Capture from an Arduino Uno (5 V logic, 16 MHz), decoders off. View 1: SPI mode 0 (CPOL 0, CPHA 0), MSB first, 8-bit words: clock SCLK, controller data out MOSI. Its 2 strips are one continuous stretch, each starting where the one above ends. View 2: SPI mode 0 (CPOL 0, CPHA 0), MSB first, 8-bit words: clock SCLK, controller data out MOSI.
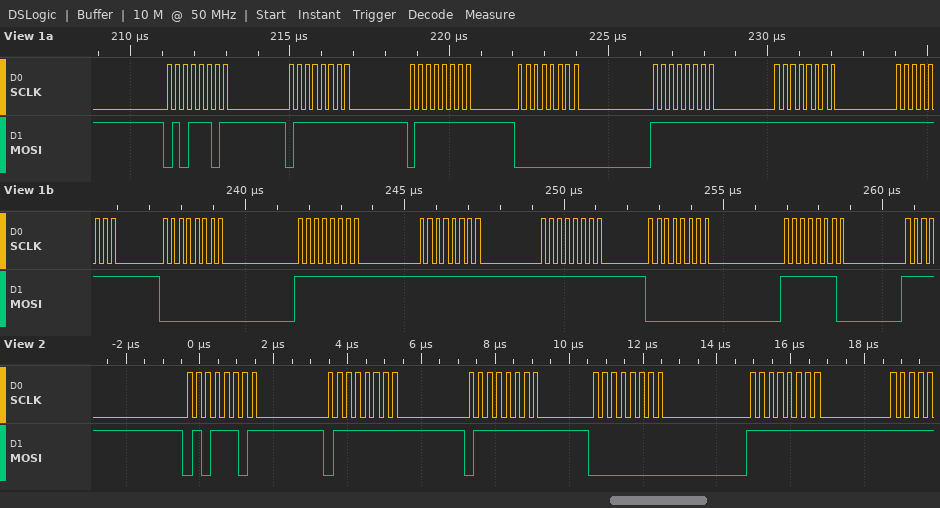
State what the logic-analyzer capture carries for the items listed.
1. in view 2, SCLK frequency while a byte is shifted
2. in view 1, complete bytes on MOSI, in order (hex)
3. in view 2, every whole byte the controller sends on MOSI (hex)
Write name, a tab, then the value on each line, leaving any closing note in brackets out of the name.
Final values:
in view 2, SCLK frequency while a byte is shifted	4 MHz
in view 1, complete bytes on MOSI, in order	0x5D 0x7F 0x7F 0x00 0xFF 0xFF 0xFF 0x00 0xFF 0xFF 0xFF 0x00 0xFE
in view 2, every whole byte the controller sends on MOSI	5D 7F 7F 00 FF
